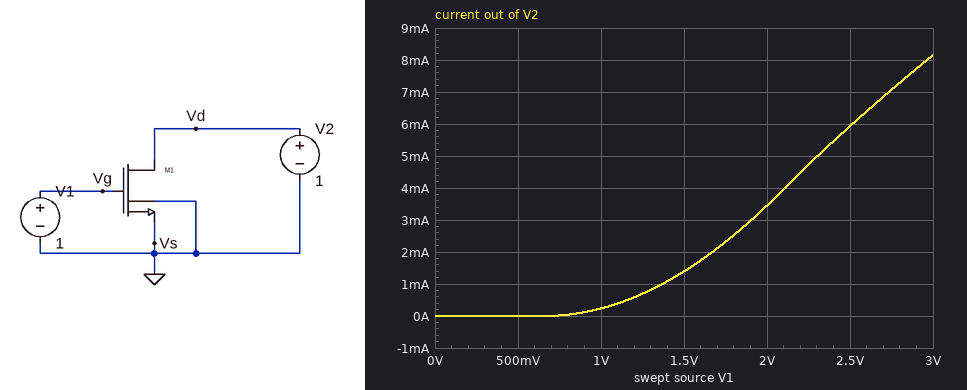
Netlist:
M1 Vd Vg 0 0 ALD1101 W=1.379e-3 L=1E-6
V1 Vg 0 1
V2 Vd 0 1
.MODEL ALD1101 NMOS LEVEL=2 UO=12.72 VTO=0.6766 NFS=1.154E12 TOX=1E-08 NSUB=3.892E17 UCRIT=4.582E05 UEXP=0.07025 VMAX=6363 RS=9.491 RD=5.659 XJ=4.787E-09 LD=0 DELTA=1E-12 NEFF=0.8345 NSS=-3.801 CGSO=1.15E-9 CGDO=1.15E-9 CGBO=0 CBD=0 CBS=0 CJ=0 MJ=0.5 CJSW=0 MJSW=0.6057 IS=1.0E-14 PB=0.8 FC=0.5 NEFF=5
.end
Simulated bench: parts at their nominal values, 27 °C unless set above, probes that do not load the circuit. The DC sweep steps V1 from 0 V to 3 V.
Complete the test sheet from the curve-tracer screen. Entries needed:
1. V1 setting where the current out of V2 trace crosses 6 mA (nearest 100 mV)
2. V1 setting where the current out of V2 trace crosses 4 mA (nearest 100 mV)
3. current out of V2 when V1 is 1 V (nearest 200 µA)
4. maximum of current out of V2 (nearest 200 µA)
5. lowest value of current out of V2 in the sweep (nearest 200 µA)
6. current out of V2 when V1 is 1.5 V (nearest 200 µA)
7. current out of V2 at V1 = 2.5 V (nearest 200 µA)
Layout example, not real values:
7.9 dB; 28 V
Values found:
2.5 V; 2.1 V; 200 µA; 8.2 mA; 0 A; 1.4 mA; 6.0 mA
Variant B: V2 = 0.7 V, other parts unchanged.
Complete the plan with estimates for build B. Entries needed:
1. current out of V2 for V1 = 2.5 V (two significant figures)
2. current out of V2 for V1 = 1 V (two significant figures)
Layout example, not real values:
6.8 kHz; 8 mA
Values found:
4.9 mA; 230 µA
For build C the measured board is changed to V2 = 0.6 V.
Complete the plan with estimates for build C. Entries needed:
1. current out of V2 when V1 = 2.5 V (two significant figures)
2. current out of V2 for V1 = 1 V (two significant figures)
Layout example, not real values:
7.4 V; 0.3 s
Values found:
4.4 mA; 230 µA
